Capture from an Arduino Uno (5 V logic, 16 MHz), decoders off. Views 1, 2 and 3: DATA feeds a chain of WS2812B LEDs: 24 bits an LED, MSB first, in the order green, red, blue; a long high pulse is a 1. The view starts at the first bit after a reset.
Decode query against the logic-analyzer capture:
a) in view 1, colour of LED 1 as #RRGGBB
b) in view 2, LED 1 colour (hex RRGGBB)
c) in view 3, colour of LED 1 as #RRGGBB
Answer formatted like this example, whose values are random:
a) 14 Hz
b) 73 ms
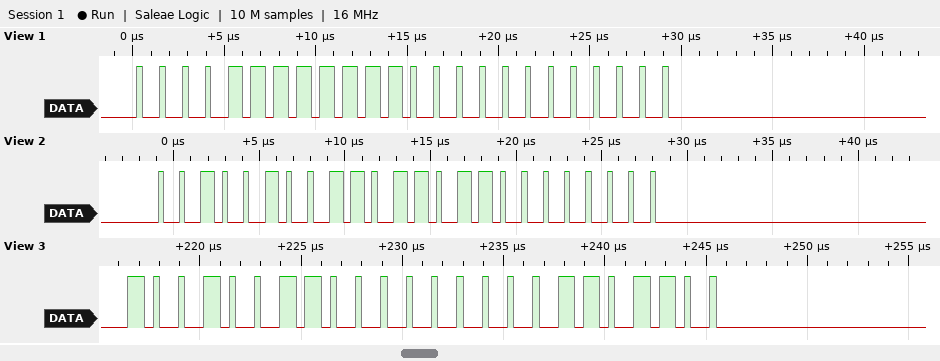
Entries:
a) #F00F00
b) #DB2400
c) #00936C
